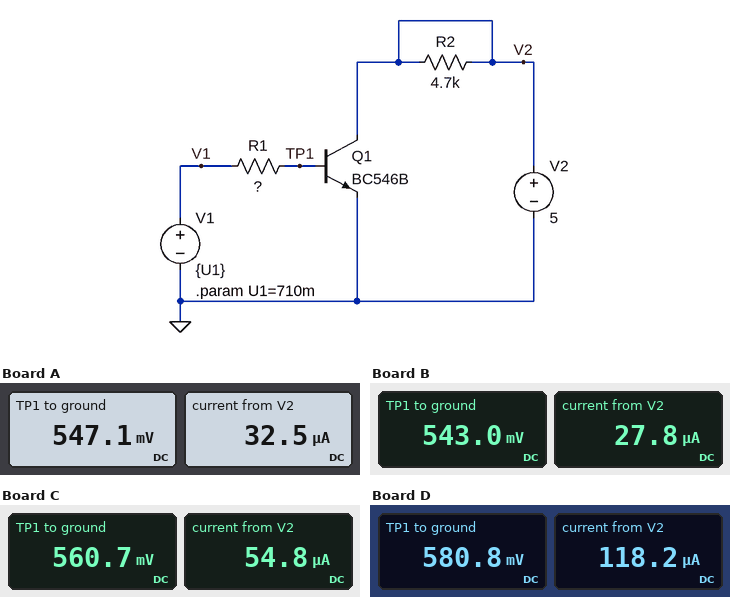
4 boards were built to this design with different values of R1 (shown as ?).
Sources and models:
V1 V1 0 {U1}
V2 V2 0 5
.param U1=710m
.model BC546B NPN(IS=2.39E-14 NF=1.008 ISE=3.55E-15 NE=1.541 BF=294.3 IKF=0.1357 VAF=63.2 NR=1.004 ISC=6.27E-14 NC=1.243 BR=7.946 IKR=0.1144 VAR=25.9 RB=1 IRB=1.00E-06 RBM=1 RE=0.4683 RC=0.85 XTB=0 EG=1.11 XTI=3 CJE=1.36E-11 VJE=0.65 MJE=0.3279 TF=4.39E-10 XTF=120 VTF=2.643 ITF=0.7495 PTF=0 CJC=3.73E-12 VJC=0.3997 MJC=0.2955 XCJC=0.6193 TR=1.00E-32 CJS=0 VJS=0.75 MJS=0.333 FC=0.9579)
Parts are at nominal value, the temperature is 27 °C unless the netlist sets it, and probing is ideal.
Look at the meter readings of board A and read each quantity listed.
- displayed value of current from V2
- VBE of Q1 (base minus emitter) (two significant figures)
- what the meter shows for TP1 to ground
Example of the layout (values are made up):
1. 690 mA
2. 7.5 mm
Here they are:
1. 32.5 µA
2. 550 mV
3. 547.1 mV
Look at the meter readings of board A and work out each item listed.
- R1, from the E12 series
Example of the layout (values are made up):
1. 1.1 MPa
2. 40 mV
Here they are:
1. 1.5 MΩ
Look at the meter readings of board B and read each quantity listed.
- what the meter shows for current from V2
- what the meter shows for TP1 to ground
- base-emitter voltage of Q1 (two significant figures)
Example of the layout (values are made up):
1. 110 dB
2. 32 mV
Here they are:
1. 27.8 µA
2. 543.0 mV
3. 540 mV
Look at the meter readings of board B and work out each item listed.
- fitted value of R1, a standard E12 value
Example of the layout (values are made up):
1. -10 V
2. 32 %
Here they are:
1. 1.8 MΩ
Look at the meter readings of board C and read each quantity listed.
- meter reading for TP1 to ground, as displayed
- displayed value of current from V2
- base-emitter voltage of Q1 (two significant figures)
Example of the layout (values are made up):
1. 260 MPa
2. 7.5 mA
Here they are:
1. 560.7 mV
2. 54.8 µA
3. 560 mV
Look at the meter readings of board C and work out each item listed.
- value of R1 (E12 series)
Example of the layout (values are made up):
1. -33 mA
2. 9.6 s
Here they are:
1. 820 kΩ
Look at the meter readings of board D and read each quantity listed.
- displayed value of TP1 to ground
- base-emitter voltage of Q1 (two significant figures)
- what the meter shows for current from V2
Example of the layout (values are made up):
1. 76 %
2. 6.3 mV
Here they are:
1. 580.8 mV
2. 580 mV
3. 118.2 µA
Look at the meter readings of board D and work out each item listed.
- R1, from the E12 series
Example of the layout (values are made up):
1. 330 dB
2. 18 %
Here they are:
1. 330 kΩ
